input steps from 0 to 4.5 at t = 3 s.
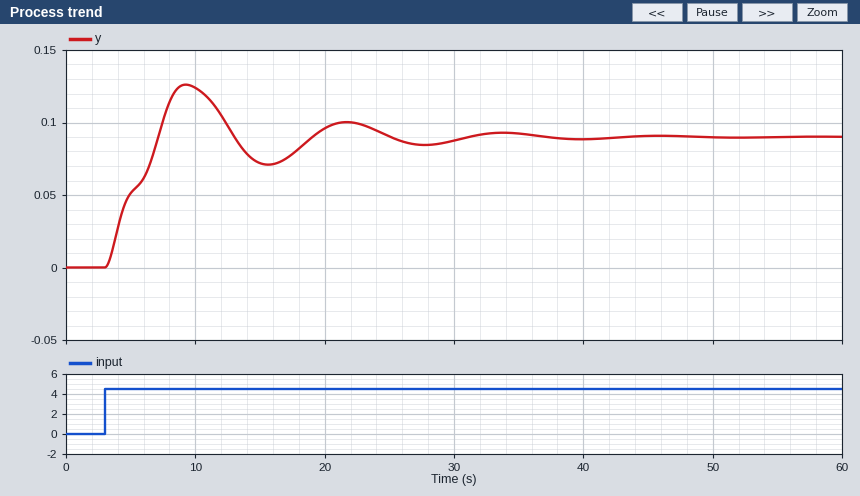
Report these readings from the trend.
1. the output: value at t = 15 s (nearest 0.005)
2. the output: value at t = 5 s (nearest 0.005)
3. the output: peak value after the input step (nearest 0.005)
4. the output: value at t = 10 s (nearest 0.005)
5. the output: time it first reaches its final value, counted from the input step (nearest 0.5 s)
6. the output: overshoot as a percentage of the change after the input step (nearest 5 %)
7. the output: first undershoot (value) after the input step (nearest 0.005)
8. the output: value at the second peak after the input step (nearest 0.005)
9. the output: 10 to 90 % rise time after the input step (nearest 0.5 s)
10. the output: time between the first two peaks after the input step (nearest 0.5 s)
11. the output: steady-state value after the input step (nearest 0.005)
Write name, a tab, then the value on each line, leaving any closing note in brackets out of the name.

the output: value at t = 15 s	0.070
the output: value at t = 5 s	0.050
the output: peak value after the input step	0.125
the output: value at t = 10 s	0.125
the output: time it first reaches its final value, counted from the input step	4.0 s
the output: overshoot as a percentage of the change after the input step	40 %
the output: first undershoot (value) after the input step	0.070
the output: value at the second peak after the input step	0.100
the output: 10 to 90 % rise time after the input step	3.5 s
the output: time between the first two peaks after the input step	12.5 s
the output: steady-state value after the input step	0.090
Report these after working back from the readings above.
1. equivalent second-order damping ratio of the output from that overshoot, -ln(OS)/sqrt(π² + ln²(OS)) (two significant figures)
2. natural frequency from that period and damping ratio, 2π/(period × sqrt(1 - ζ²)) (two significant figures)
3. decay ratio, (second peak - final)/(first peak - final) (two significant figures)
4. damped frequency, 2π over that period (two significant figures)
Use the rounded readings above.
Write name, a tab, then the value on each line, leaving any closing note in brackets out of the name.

equivalent second-order damping ratio of the output from that overshoot, -ln(OS)/sqrt(π² + ln²(OS))	0.28
natural frequency from that period and damping ratio, 2π/(period × sqrt(1 - ζ²))	0.52 rad/s
decay ratio, (second peak - final)/(first peak - final)	0.29
damped frequency, 2π over that period	0.50 rad/s
